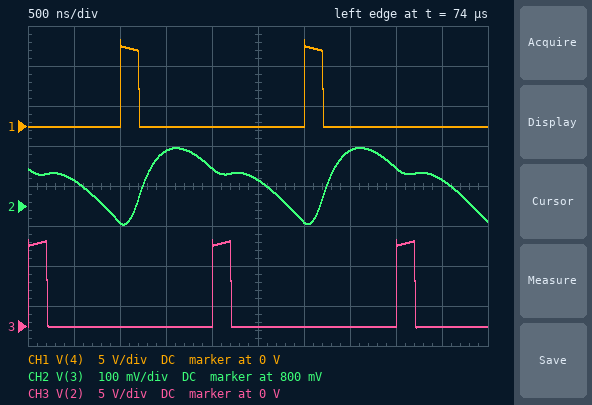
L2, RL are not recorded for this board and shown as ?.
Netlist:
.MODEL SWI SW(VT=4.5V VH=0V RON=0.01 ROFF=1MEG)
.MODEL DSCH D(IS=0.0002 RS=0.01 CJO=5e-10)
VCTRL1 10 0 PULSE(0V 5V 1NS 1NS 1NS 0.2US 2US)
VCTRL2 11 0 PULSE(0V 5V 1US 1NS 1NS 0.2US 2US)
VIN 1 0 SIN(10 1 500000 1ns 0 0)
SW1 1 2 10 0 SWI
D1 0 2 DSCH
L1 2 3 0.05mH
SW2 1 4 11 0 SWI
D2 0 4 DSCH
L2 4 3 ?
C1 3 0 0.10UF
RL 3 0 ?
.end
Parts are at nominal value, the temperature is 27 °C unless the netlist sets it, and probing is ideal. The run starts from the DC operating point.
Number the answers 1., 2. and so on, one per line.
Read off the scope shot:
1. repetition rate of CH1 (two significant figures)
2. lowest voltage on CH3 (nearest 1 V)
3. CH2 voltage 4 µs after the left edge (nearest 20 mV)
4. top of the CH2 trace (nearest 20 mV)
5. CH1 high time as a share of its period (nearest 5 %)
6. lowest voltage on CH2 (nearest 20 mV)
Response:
1. 500 kHz
2. 0 V
3. 900 mV
4. 940 mV
5. 10 %
6. 760 mV
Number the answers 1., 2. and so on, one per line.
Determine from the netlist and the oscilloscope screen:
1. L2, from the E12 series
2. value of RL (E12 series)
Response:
1. 15 µH
2. 3.3 Ω
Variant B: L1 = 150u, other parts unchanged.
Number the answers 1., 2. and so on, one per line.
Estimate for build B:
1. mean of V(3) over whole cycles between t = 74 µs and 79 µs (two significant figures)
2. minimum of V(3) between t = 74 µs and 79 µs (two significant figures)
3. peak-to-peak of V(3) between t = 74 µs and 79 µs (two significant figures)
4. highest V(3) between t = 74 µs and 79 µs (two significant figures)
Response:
1. 840 mV
2. 720 mV
3. 210 mV
4. 930 mV
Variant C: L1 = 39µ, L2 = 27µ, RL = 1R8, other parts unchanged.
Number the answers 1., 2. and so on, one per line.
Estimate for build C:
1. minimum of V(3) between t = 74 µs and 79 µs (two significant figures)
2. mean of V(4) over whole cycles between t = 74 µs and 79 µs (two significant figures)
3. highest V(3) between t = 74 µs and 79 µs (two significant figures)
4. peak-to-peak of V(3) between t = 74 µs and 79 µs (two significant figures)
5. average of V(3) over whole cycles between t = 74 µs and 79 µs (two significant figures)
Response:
1. 810 mV
2. 830 mV
3. 880 mV
4. 65 mV
5. 850 mV
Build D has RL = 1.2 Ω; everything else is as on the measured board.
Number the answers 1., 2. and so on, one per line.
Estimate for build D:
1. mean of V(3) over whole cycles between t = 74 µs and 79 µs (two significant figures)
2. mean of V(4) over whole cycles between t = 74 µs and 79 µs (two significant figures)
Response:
1. 820 mV
2. 800 mV
